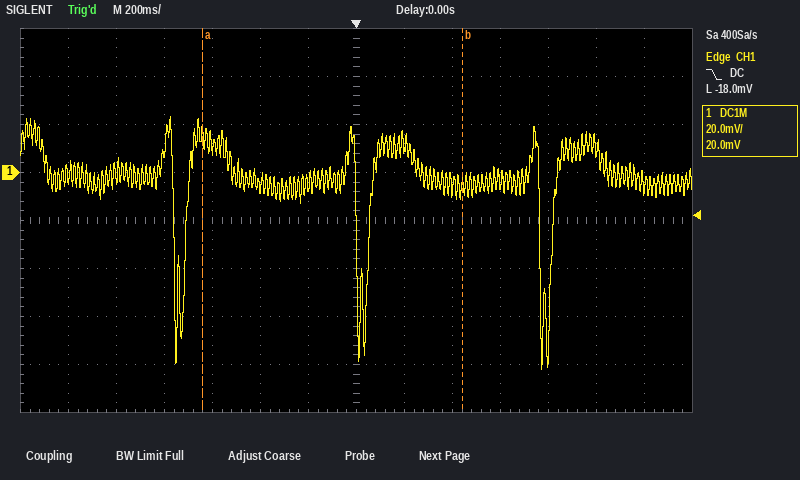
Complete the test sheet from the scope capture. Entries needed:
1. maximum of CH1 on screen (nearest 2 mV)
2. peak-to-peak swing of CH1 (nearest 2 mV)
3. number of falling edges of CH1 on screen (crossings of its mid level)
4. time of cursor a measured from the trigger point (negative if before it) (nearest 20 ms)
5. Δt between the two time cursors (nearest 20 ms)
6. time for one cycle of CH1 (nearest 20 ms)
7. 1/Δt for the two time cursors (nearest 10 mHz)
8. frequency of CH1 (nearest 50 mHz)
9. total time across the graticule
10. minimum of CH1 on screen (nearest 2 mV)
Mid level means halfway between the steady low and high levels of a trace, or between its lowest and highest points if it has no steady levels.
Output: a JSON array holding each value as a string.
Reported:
["24 mV", "106 mV", "3", "-640 ms", "1.08 s", "760 ms", "930 mHz", "1.30 Hz", "2.8 s", "-82 mV"]
